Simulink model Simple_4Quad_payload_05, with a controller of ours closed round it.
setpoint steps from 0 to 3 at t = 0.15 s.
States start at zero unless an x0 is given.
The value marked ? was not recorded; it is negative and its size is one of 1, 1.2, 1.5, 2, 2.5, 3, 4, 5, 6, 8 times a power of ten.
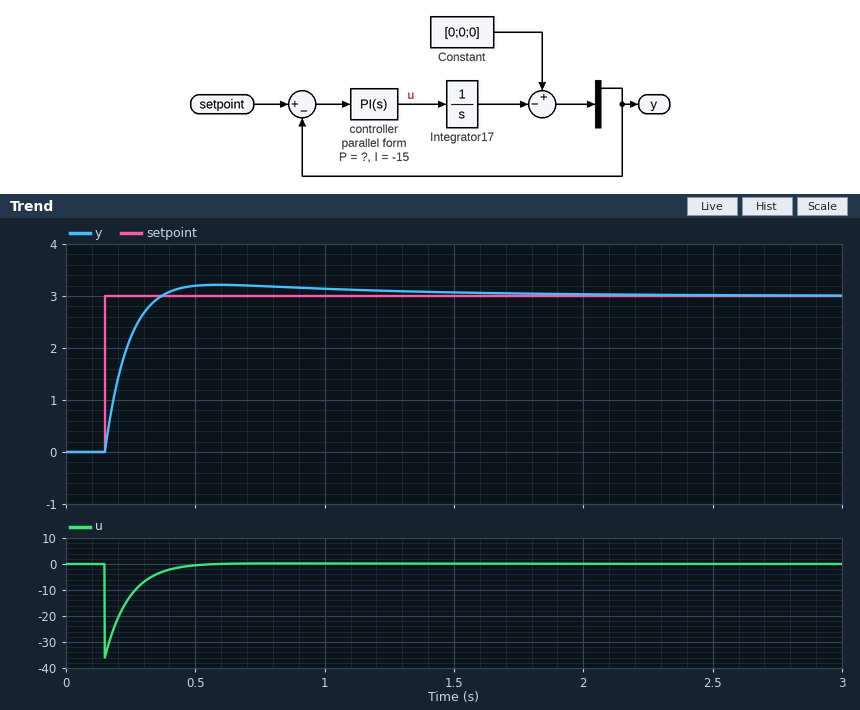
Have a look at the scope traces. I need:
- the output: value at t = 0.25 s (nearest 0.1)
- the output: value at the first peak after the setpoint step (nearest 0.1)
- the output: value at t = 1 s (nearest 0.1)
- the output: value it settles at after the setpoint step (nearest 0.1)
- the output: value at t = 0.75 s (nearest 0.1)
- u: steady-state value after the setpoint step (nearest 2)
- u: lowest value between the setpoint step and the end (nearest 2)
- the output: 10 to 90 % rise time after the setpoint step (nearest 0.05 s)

2.2
3.2
3.1
3.0
3.2
0
-36
0.15 s
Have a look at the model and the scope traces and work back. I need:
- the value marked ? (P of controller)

-12
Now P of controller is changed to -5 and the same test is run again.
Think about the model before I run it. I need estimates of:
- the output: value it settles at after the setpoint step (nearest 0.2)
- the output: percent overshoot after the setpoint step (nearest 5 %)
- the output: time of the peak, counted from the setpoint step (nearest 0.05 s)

3.0
25 %
0.60 s
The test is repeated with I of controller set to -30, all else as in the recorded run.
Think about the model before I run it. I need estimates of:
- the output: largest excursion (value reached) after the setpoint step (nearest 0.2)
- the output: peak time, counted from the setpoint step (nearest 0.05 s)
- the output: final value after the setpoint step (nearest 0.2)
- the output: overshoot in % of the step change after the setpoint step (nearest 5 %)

3.4
0.35 s
3.0
10 %
